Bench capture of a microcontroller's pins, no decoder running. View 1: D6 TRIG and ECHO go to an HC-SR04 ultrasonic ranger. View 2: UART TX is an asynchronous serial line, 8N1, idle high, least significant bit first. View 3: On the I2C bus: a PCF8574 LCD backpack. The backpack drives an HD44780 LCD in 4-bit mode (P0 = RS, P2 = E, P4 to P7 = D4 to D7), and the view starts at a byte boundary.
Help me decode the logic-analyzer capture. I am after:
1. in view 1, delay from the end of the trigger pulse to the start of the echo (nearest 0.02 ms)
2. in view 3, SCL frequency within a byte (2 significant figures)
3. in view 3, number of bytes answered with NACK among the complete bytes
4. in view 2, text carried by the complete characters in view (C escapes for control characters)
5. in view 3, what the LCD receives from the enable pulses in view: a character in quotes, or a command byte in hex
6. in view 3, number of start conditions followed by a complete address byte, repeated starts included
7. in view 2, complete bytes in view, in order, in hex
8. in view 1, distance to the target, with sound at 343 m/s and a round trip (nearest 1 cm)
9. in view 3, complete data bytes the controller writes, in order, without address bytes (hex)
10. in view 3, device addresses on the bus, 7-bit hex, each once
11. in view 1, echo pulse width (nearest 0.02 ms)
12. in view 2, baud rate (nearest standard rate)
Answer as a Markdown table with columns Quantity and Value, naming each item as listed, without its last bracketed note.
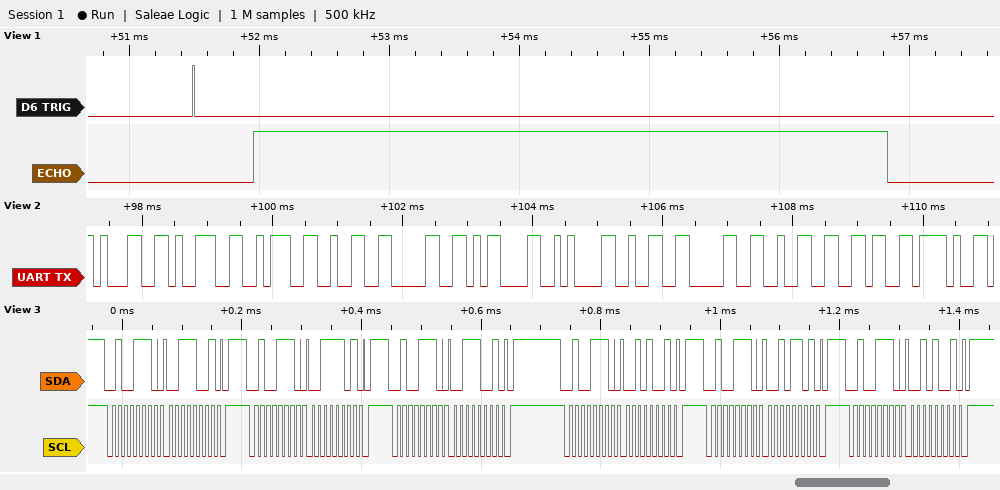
| Quantity | Value |
|---|---|
| in view 1, delay from the end of the trigger pulse to the start of the echo | 0.46 ms |
| in view 3, SCL frequency within a byte | 100 kHz |
| in view 3, number of bytes answered with NACK among the complete bytes | 0 |
| in view 2, text carried by the complete characters in view | "19:20\r\n2026/" |
| in view 3, what the LCD receives from the enable pulses in view: a character in quotes, or a command byte in hex | '2' |
| in view 3, number of start conditions followed by a complete address byte, repeated starts included | 6 |
| in view 2, complete bytes in view, in order, in hex | 0x31 0x39 0x3A 0x32 0x30 0x0D 0x0A 0x32 0x30 0x32 0x36 0x2F |
| in view 1, distance to the target, with sound at 343 m/s and a round trip | 84 cm |
| in view 3, complete data bytes the controller writes, in order, without address bytes | 39 3D 39 29 2D 29 |
| in view 3, device addresses on the bus, 7-bit hex, each once | 0x27 |
| in view 1, echo pulse width | 4.88 ms |
| in view 2, baud rate | 9600 baud |
